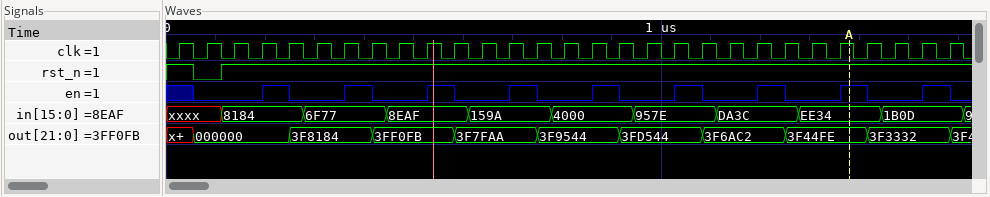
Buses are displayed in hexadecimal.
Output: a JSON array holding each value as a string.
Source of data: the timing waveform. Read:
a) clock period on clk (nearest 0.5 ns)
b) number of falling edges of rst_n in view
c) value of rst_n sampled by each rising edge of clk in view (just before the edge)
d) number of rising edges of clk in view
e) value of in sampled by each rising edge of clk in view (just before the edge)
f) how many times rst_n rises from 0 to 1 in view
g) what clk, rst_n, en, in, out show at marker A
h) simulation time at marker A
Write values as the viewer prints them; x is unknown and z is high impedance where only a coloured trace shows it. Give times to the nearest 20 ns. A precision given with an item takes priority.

["55.5 ns", "1", "1 0 1 1 1 1 1 1 1 1 1 1 1 1 1 1 1 1 1 1 1 1 1 1 1 1 1 1 1", "29", "xxxx, xxxx, 8184, 8184, 8184, 6F77, 6F77, 6F77, 8EAF, 8EAF, 8EAF, 159A, 159A, 159A, 4000, 4000, 4000, 957E, 957E, 957E, DA3C, DA3C, DA3C, EE34, EE34, EE34, 1B0D, 1B0D, 1B0D", "1", "clk=1, rst_n=1, en=1, in=EE34, out=3F44FE", "1380 ns"]
